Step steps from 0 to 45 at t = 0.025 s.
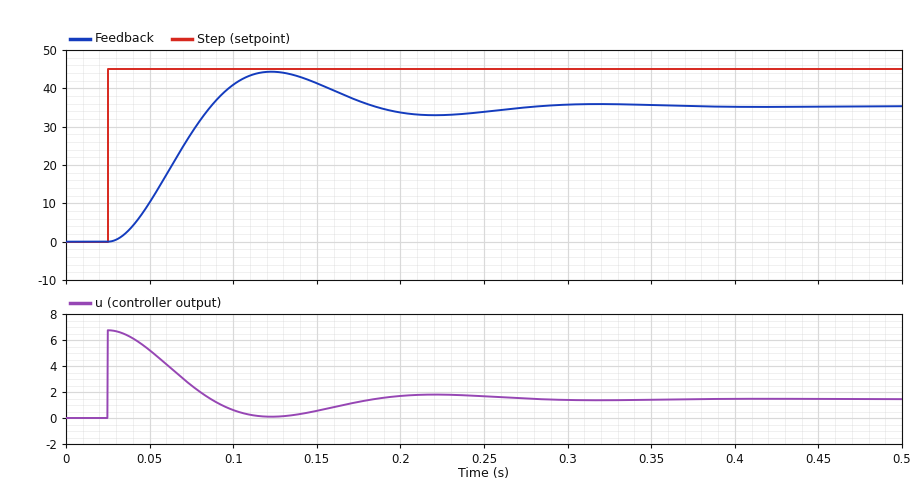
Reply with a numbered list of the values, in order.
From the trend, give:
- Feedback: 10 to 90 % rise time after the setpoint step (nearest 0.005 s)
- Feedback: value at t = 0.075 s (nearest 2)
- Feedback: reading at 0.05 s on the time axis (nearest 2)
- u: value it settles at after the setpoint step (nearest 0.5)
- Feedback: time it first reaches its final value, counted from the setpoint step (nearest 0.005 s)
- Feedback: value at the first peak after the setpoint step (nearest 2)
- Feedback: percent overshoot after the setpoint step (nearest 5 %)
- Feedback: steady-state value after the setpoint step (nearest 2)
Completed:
1. 0.040 s
2. 28
3. 10
4. 1.5
5. 0.060 s
6. 44
7. 25 %
8. 36
